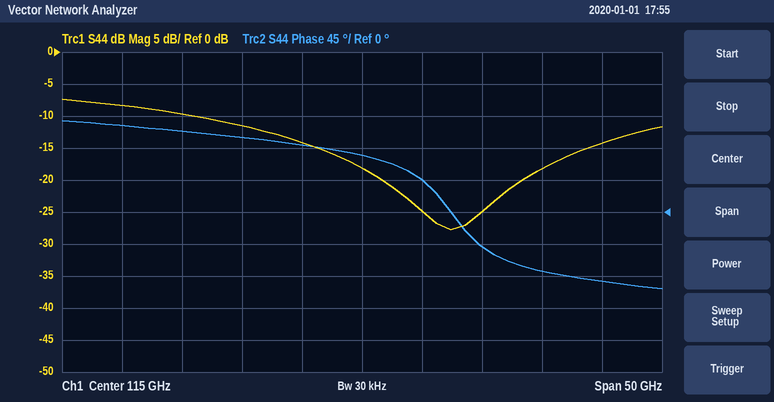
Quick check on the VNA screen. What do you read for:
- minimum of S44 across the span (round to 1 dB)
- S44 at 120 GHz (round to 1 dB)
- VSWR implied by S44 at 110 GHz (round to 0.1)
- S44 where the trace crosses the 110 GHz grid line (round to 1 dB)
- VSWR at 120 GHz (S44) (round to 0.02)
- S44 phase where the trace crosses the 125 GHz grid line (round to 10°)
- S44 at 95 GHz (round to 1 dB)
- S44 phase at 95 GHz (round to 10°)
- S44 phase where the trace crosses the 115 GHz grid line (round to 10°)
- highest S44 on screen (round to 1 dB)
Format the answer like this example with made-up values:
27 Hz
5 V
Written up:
-28 dB
-25 dB
1.5
-14 dB
1.12
-50°
-8 dB
120°
80°
-7 dB
